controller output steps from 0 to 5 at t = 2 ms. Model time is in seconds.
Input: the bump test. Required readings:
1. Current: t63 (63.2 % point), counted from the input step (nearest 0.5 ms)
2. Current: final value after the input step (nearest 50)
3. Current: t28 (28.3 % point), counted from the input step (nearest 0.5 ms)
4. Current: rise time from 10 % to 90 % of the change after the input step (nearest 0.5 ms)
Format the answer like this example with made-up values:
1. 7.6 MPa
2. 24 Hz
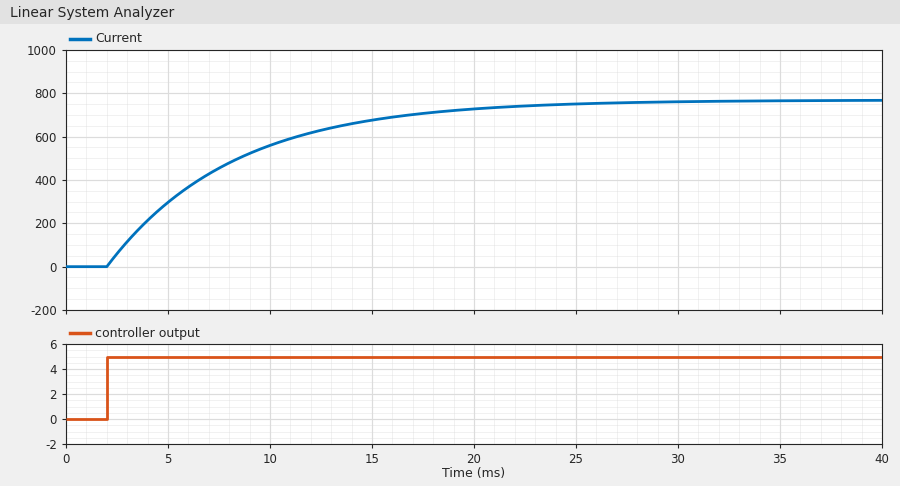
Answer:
1. 6.0 ms
2. 750
3. 2.0 ms
4. 13.5 ms
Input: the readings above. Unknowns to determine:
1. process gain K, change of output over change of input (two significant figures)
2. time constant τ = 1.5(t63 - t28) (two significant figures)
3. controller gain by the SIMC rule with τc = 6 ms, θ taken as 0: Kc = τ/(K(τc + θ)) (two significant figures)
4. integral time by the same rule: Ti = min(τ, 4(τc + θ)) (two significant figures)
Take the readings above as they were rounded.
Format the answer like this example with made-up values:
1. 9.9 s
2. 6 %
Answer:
1. 150
2. 6.0 ms
3. 0.0067
4. 6.0 ms
